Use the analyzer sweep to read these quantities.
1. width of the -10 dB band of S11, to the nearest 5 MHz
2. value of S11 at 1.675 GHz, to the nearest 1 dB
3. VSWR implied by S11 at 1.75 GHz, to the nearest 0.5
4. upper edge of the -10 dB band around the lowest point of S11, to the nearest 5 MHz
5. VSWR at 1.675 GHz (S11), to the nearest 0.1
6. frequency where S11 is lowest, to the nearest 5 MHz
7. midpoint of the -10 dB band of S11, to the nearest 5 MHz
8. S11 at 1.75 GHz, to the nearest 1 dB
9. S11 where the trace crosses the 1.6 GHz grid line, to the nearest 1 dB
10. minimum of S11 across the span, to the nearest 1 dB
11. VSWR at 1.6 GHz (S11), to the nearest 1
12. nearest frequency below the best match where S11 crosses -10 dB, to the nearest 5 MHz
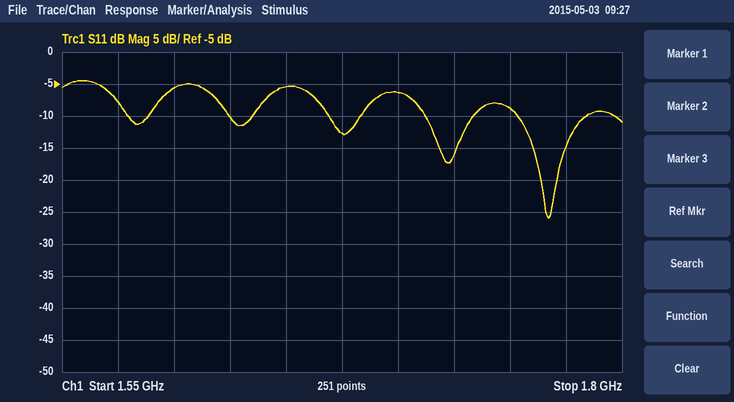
30 MHz
-13 dB
2.0
1.785 GHz
1.6
1.765 GHz
1.770 GHz
-9 dB
-6 dB
-26 dB
3
1.755 GHz
